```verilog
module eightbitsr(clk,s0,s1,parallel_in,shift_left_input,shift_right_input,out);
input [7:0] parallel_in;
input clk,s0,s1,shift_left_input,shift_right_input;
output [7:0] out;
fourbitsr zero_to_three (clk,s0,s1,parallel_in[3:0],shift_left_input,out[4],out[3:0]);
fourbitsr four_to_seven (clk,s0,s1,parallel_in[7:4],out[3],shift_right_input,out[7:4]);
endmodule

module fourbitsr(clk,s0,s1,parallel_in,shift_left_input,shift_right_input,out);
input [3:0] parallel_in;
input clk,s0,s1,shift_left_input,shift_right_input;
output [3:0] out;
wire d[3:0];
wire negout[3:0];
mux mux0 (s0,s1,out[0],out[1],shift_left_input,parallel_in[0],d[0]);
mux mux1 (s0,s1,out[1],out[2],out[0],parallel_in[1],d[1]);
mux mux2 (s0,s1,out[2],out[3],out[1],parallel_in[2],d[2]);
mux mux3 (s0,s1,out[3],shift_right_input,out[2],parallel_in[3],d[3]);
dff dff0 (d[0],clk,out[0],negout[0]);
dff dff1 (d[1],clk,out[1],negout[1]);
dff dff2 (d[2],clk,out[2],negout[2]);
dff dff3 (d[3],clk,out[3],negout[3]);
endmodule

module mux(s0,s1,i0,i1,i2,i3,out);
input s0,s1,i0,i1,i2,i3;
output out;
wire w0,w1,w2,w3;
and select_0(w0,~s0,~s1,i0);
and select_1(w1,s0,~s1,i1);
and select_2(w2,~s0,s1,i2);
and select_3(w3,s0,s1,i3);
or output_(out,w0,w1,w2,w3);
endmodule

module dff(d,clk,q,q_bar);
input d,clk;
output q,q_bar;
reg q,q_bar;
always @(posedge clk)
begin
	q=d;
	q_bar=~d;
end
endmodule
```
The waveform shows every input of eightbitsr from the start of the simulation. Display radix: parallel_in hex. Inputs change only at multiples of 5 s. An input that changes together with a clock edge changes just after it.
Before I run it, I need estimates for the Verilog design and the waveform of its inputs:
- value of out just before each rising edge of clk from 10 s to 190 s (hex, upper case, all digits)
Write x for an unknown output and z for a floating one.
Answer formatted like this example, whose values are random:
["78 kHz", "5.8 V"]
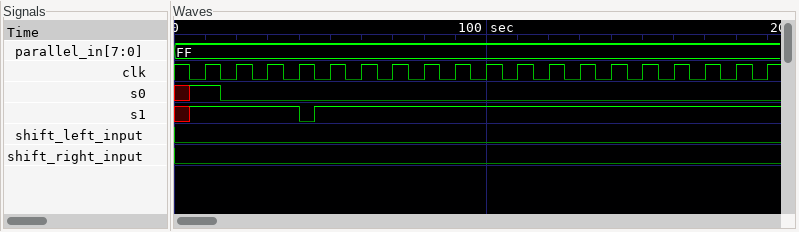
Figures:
["x, FF, FE, FC, F8, F0, E0, C0, 80, 00, 00, 00, 00, 00, 00, 00, 00, 00, 00"]
